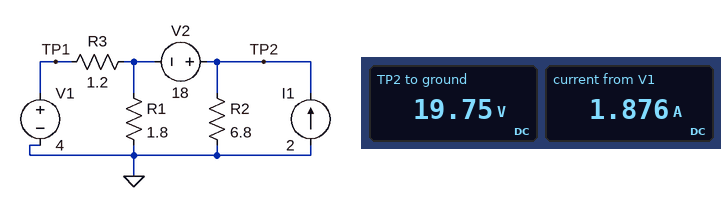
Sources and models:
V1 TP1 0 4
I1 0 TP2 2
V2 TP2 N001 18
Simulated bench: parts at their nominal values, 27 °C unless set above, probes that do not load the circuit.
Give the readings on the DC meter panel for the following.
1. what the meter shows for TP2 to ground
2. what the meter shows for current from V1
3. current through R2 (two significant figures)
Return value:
19.75 V
1.876 A
2.9 A
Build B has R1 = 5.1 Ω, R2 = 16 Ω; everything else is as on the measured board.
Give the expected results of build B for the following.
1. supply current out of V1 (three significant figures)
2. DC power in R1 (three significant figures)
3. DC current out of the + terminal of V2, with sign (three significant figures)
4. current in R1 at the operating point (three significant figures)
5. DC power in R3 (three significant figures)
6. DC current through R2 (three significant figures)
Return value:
122 mA
2.91 W
-634 mA
756 mA
17.7 mW
1.37 A
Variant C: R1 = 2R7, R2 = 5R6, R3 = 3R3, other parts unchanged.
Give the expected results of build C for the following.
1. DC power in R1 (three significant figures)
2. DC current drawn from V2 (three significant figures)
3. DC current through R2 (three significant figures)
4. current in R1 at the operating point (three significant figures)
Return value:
2.39 µW
1.21 A
3.21 A
941 µA
